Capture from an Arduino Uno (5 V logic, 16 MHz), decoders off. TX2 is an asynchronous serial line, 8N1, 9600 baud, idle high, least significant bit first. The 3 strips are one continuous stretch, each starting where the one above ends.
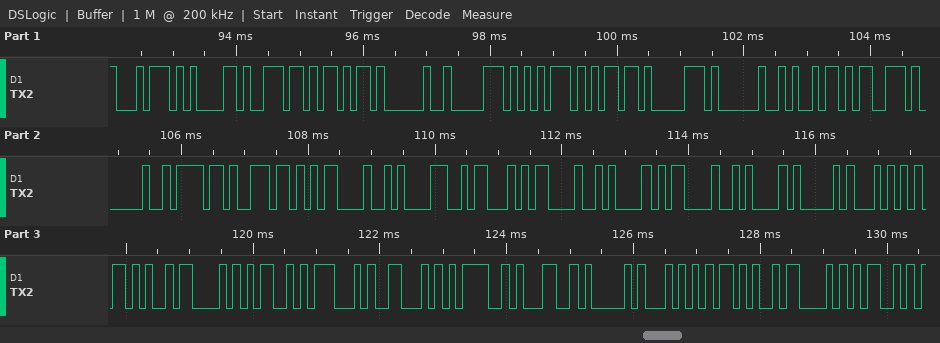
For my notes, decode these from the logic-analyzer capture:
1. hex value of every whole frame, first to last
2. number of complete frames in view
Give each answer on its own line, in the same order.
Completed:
0x74 0x61 0x6E 0x6B 0x20 0x70 0x75 0x6D 0x70 0x20 0x69 0x73 0x20 0x6F 0x6E 0x0D 0x0A 0x1A 0x0D 0x0A 0x0D 0x0A 0x41 0x54 0x2B 0x43 0x4D 0x47 0x46 0x3D 0x31 0x41 0x54 0x2B 0x43 0x4D
36
